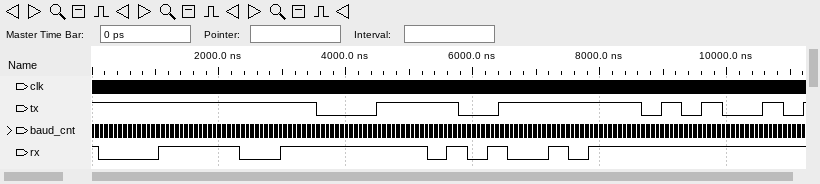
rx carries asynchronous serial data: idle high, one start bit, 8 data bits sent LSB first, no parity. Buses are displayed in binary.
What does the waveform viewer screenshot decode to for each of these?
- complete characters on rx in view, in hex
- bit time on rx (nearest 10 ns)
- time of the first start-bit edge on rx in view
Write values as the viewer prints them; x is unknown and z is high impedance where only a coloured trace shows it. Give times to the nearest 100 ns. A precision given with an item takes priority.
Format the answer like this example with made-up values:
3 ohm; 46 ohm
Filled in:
3C, A5; 310 ns; 100 ns
